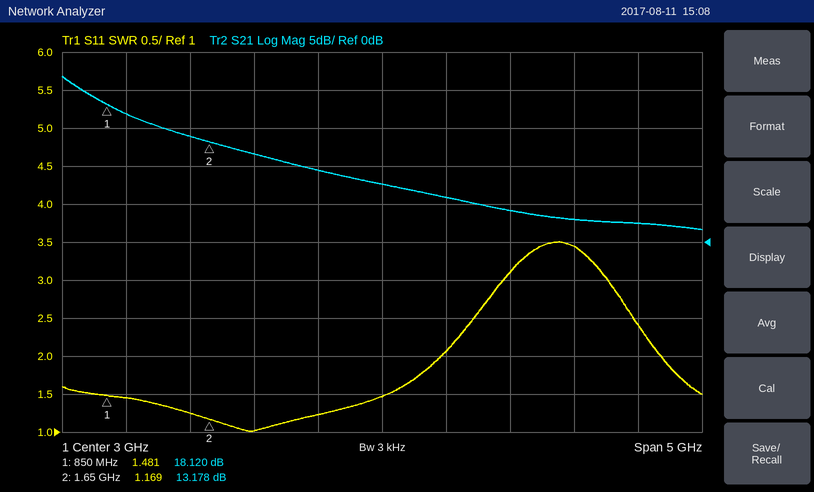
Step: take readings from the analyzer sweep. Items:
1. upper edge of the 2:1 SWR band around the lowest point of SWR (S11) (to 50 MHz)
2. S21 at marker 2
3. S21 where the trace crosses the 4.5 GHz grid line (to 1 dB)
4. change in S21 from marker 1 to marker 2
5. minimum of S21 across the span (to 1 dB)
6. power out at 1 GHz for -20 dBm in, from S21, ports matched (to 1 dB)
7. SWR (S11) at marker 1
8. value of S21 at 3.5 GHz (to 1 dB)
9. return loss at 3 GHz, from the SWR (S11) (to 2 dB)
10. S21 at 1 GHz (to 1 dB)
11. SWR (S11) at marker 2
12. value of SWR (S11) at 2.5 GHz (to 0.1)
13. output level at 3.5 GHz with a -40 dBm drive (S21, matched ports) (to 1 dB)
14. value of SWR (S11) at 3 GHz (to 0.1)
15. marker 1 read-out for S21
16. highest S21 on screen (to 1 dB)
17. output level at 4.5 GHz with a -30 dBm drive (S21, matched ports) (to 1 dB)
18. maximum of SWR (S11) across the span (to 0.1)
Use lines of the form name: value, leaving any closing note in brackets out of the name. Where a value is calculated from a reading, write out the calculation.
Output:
upper edge of the 2:1 SWR band around the lowest point of SWR (S11): 3.45 GHz
S21 at marker 2: 13.178 dB
S21 where the trace crosses the 4.5 GHz grid line: 3 dB
change in S21 from marker 1 to marker 2: 13.178 − (18.12) = -4.942 dB
minimum of S21 across the span: 2 dB
power out at 1 GHz for -20 dBm in, from S21, ports matched: -20 dBm + (17 dB) = -3 dBm
SWR (S11) at marker 1: 1.481
value of S21 at 3.5 GHz: 6 dB
return loss at 3 GHz, from the SWR (S11): −20 log10((1.5 − 1)/(1.5 + 1)) ≈ 14 dB
S21 at 1 GHz: 17 dB
SWR (S11) at marker 2: 1.169
value of SWR (S11) at 2.5 GHz: 1.2
output level at 3.5 GHz with a -40 dBm drive (S21, matched ports): -40 dBm + (6 dB) = -34 dBm
value of SWR (S11) at 3 GHz: 1.5
marker 1 read-out for S21: 18.120 dB
highest S21 on screen: 22 dB
output level at 4.5 GHz with a -30 dBm drive (S21, matched ports): -30 dBm + (3 dB) = -27 dBm
maximum of SWR (S11) across the span: 3.5
